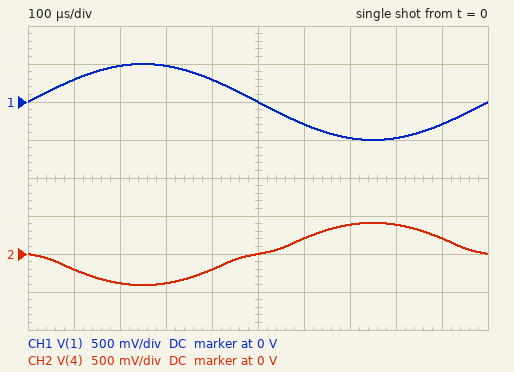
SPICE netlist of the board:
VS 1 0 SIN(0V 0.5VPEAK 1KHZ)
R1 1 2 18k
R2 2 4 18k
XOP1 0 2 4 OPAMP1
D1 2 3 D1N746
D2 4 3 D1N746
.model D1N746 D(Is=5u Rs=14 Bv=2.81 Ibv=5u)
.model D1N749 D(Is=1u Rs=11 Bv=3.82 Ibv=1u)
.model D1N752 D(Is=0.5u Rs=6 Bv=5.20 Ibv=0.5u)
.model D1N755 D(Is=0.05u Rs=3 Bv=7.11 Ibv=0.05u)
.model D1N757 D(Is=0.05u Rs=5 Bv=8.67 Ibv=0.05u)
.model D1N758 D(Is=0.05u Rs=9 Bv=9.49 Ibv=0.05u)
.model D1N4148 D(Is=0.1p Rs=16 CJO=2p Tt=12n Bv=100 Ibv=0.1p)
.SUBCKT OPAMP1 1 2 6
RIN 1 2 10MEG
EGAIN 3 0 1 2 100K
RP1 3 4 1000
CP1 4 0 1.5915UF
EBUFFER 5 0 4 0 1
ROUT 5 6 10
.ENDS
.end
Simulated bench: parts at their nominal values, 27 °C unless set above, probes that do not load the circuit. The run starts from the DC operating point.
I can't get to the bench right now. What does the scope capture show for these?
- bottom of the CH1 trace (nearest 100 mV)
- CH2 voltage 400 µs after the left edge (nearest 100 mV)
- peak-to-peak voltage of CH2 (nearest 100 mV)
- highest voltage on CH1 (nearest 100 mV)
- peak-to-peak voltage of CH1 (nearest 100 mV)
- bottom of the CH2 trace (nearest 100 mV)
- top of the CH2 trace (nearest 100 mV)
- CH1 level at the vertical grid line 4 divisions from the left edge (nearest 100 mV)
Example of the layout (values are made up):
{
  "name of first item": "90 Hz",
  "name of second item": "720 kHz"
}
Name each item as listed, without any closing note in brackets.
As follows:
{
  "bottom of the CH1 trace": "-500 mV",
  "CH2 voltage 400 µs after the left edge": "-200 mV",
  "peak-to-peak voltage of CH2": "800 mV",
  "highest voltage on CH1": "500 mV",
  "peak-to-peak voltage of CH1": "1.0 V",
  "bottom of the CH2 trace": "-400 mV",
  "top of the CH2 trace": "400 mV",
  "CH1 level at the vertical grid line 4 divisions from the left edge": "300 mV"
}
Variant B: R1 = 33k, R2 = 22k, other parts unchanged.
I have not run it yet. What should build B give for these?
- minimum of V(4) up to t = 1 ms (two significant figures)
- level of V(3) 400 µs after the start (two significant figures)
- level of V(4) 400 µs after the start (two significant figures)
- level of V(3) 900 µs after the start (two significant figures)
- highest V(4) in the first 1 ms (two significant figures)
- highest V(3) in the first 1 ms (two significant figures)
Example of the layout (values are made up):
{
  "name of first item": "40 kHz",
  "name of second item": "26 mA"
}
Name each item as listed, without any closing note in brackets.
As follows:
{
  "minimum of V(4) up to t = 1 ms": "-220 mV",
  "level of V(3) 400 µs after the start": "-17 mV",
  "level of V(4) 400 µs after the start": "-92 mV",
  "level of V(3) 900 µs after the start": "75 mV",
  "highest V(4) in the first 1 ms": "220 mV",
  "highest V(3) in the first 1 ms": "210 mV"
}
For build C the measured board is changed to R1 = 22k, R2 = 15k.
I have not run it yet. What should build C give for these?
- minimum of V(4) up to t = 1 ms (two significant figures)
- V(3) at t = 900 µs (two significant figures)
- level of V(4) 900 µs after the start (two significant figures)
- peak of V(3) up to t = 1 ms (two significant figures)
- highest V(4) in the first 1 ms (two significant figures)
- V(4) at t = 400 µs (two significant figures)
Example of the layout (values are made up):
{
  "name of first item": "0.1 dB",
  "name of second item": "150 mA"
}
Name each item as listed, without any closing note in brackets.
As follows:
{
  "minimum of V(4) up to t = 1 ms": "-270 mV",
  "V(3) at t = 900 µs": "110 mV",
  "level of V(4) 900 µs after the start": "130 mV",
  "peak of V(3) up to t = 1 ms": "250 mV",
  "highest V(4) in the first 1 ms": "270 mV",
  "V(4) at t = 400 µs": "-130 mV"
}
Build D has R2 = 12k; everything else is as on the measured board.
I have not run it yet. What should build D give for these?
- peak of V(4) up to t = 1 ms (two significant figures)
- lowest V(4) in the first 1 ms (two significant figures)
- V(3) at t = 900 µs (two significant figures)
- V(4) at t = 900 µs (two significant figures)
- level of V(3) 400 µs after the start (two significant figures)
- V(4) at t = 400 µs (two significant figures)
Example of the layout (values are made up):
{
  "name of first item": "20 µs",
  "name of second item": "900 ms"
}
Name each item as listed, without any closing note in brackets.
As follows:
{
  "peak of V(4) up to t = 1 ms": "270 mV",
  "lowest V(4) in the first 1 ms": "-270 mV",
  "V(3) at t = 900 µs": "120 mV",
  "V(4) at t = 900 µs": "140 mV",
  "level of V(3) 400 µs after the start": "-18 mV",
  "V(4) at t = 400 µs": "-140 mV"
}
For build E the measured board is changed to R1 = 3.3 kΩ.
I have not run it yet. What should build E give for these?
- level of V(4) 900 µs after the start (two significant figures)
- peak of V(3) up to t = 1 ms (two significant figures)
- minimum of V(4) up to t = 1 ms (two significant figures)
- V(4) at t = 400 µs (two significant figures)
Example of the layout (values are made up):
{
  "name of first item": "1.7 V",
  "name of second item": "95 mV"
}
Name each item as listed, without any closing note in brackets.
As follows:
{
  "level of V(4) 900 µs after the start": "1.5 V",
  "peak of V(3) up to t = 1 ms": "2.6 V",
  "minimum of V(4) up to t = 1 ms": "-2.6 V",
  "V(4) at t = 400 µs": "-1.5 V"
}
